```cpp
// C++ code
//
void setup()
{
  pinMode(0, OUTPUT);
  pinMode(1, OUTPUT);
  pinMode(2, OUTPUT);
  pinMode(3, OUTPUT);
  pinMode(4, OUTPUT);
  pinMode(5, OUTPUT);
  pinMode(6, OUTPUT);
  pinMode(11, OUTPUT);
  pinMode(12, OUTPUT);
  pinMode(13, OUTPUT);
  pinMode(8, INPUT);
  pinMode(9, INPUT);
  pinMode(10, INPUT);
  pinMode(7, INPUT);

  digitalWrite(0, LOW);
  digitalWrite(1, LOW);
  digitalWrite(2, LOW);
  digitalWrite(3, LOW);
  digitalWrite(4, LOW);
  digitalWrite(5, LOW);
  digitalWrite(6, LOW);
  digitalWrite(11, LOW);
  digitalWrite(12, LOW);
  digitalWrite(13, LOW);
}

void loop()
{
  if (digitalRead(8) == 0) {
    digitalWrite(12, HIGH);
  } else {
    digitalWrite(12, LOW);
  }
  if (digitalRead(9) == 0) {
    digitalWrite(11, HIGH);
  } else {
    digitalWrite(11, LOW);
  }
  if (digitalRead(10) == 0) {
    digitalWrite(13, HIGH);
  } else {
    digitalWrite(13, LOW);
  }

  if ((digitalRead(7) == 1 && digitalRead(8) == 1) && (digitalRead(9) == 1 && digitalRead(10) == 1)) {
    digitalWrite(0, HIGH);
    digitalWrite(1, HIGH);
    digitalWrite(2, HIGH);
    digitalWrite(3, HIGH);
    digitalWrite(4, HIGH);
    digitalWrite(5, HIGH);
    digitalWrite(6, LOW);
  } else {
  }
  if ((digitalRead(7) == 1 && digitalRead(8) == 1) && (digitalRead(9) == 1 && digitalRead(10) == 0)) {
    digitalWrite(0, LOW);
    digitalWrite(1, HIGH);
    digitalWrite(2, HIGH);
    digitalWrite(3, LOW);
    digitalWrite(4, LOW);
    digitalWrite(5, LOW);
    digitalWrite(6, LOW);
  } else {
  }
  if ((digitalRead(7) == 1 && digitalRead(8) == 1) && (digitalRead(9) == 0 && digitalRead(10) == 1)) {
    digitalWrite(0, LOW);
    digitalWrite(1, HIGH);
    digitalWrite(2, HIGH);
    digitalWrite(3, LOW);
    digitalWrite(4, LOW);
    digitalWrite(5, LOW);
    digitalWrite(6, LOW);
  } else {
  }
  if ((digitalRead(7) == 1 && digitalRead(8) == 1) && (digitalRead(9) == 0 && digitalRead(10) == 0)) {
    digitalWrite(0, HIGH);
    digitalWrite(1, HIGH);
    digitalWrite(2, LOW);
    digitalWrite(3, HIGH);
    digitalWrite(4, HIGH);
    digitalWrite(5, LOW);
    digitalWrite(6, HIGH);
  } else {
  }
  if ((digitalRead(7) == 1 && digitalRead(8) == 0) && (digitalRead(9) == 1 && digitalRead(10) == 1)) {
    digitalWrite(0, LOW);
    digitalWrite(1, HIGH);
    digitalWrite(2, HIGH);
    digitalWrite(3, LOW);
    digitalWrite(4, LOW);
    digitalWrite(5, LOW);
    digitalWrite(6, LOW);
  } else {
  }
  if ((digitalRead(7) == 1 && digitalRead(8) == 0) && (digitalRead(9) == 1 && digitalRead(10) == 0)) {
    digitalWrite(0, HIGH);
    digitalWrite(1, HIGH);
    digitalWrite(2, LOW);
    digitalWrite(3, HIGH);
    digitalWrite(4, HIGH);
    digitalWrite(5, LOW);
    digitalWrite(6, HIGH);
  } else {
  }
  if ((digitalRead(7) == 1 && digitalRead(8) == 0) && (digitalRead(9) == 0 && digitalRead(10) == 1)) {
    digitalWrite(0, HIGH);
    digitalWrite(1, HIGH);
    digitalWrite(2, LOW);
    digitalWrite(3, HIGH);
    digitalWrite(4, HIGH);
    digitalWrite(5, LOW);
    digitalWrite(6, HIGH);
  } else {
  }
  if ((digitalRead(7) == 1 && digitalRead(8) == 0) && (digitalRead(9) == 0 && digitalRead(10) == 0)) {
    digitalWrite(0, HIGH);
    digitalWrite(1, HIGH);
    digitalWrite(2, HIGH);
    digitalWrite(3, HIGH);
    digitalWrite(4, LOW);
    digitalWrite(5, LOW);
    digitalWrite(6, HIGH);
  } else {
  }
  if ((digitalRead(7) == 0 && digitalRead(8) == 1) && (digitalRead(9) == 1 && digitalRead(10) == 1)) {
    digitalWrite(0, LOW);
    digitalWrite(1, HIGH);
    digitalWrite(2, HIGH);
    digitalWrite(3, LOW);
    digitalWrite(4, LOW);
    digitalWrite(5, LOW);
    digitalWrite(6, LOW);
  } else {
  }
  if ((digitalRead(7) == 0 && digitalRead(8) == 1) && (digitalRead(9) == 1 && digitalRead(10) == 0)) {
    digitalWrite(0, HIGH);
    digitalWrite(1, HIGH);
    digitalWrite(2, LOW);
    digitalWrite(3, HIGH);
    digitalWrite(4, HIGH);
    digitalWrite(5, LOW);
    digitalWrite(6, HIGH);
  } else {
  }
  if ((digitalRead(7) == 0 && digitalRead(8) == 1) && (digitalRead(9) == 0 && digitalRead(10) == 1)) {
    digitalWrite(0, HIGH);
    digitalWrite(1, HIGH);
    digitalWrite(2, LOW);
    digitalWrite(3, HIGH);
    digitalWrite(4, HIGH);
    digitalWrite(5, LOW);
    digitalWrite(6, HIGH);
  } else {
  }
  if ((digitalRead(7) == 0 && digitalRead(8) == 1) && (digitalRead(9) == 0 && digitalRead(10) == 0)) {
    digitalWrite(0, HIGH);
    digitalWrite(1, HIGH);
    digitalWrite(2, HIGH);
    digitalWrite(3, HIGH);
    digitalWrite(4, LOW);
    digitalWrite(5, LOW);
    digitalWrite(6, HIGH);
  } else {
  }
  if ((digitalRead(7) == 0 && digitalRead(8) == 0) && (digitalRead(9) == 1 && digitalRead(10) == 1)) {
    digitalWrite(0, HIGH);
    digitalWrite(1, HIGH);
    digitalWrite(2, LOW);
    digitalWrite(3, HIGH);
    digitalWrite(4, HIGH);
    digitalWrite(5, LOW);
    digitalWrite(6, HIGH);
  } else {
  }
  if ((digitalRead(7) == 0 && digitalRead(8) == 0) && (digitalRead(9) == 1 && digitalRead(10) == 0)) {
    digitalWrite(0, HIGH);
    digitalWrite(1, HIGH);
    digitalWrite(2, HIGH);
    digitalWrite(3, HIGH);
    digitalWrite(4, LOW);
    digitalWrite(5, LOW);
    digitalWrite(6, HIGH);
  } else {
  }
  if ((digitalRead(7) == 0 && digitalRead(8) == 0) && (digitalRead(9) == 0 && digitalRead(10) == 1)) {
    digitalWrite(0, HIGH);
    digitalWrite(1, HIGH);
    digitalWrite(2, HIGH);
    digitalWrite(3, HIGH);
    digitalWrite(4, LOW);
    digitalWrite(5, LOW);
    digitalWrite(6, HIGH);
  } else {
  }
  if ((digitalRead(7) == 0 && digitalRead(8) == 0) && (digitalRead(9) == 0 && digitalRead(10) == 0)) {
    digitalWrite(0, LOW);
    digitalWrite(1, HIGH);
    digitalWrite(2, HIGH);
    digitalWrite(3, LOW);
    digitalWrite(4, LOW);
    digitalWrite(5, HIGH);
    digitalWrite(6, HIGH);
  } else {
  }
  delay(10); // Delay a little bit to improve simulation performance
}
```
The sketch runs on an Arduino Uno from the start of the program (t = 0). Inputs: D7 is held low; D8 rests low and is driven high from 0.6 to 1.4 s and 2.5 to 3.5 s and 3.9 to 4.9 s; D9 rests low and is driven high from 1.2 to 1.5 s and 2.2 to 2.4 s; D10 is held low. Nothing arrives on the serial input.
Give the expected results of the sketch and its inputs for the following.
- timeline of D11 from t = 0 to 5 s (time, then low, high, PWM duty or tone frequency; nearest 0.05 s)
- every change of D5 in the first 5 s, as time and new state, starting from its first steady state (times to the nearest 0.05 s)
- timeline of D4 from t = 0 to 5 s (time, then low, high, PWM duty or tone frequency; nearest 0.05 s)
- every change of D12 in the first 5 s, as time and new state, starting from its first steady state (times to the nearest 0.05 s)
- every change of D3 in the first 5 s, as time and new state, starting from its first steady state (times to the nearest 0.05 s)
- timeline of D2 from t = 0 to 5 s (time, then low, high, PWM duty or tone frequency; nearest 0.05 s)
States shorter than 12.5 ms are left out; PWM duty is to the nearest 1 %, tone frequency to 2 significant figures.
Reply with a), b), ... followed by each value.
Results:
a) 0 s high; 1.2 s low; 1.5 s high; 2.2 s low; 2.4 s high
b) 0 s high; 0.6 s low; 1.5 s high; 2.2 s low; 2.4 s high; 2.5 s low; 3.5 s high; 3.9 s low; 4.9 s high
c) 0 s low; 1.2 s high; 1.4 s low
d) 0 s high; 0.6 s low; 1.4 s high; 2.5 s low; 3.5 s high; 3.9 s low; 4.9 s high
e) 0 s low; 0.6 s high; 1.5 s low; 2.2 s high; 2.4 s low; 2.5 s high; 3.5 s low; 3.9 s high; 4.9 s low
f) 0 s high; 1.2 s low; 1.4 s high
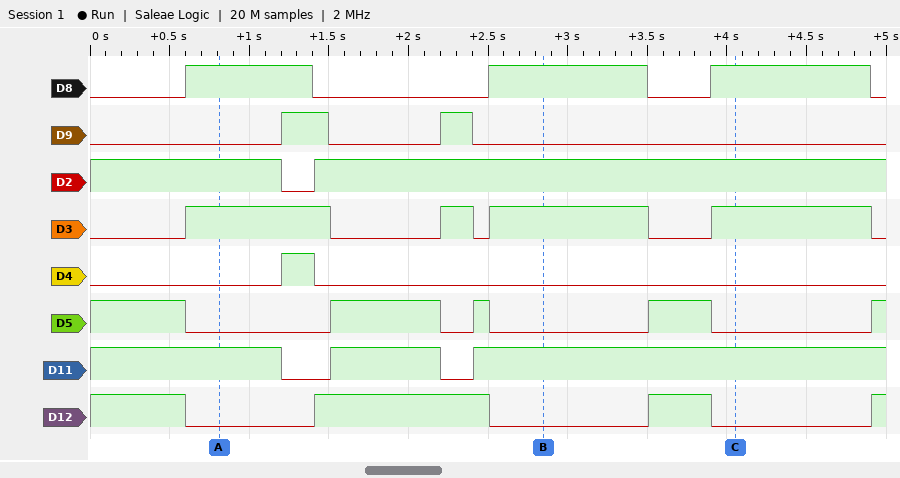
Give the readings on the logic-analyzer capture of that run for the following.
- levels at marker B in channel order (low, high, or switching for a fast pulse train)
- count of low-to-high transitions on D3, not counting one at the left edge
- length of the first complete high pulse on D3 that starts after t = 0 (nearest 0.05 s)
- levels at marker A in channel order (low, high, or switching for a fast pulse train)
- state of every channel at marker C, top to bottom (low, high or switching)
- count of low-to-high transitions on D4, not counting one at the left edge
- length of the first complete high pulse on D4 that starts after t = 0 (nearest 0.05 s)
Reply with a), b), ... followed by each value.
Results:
a) D8 high, D9 low, D2 high, D3 high, D4 low, D5 low, D11 high, D12 low
b) 4
c) 0.90 s
d) D8 high, D9 low, D2 high, D3 high, D4 low, D5 low, D11 high, D12 low
e) D8 high, D9 low, D2 high, D3 high, D4 low, D5 low, D11 high, D12 low
f) 1
g) 0.20 s
